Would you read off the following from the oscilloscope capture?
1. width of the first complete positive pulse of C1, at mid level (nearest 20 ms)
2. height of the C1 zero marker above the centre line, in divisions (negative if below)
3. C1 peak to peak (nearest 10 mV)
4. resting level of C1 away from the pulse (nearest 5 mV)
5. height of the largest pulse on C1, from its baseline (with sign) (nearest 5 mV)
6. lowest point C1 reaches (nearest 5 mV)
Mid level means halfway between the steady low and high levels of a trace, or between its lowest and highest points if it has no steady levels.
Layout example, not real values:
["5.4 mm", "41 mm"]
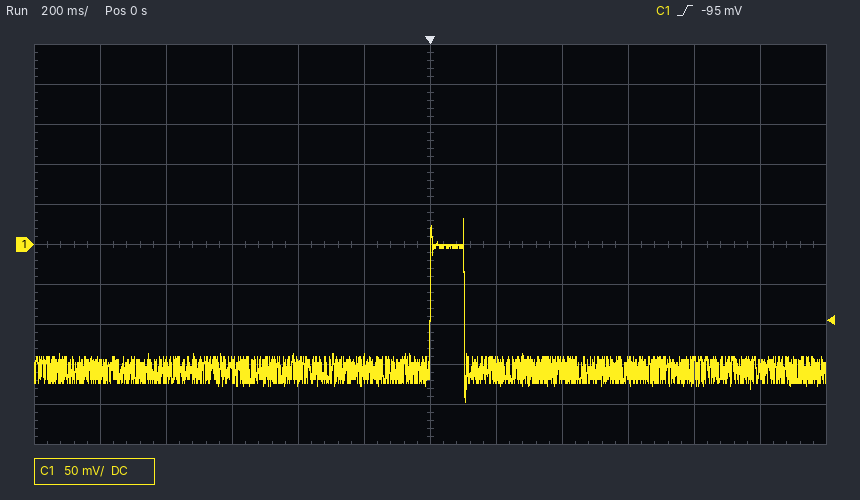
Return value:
["100 ms", "0.0 div", "230 mV", "-155 mV", "+190 mV", "-195 mV"]
